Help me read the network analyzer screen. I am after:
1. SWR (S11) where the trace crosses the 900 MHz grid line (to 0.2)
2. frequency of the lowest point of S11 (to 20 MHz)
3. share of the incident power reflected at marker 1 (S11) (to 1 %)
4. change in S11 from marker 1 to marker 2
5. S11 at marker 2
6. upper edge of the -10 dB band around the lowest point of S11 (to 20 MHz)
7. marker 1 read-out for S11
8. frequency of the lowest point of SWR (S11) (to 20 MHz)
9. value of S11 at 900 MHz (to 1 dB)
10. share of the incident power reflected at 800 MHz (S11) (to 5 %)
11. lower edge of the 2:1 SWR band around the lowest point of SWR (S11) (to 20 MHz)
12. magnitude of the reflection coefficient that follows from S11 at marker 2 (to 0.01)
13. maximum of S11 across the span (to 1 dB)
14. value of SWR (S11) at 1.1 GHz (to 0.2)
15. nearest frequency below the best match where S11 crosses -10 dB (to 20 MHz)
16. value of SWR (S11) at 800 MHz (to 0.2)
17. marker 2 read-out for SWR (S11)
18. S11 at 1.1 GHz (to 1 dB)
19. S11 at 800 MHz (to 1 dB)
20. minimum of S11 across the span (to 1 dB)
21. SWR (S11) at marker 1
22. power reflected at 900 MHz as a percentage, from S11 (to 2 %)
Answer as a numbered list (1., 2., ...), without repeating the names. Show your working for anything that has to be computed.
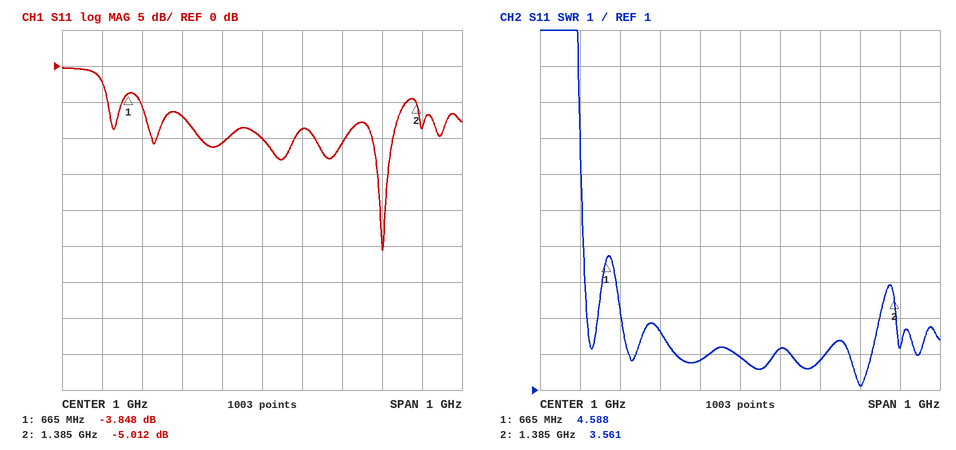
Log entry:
1. 1.8
2. 1.30 GHz
3. 10^(-3.848/10) ≈ 41 %
4. -5.012 − (-3.848) = -1.164 dB
5. -5.012 dB
6. 1.32 GHz
7. -3.848 dB
8. 1.30 GHz
9. -11 dB
10. 10^(-7/10) ≈ 20 %
11. 1.28 GHz
12. 10^(-5.012/20) ≈ 0.56
13. 0 dB
14. 2.2
15. 1.28 GHz
16. 2.6
17. 3.561
18. -9 dB
19. -7 dB
20. -26 dB
21. 4.588
22. 10^(-11/10) ≈ 8 %
